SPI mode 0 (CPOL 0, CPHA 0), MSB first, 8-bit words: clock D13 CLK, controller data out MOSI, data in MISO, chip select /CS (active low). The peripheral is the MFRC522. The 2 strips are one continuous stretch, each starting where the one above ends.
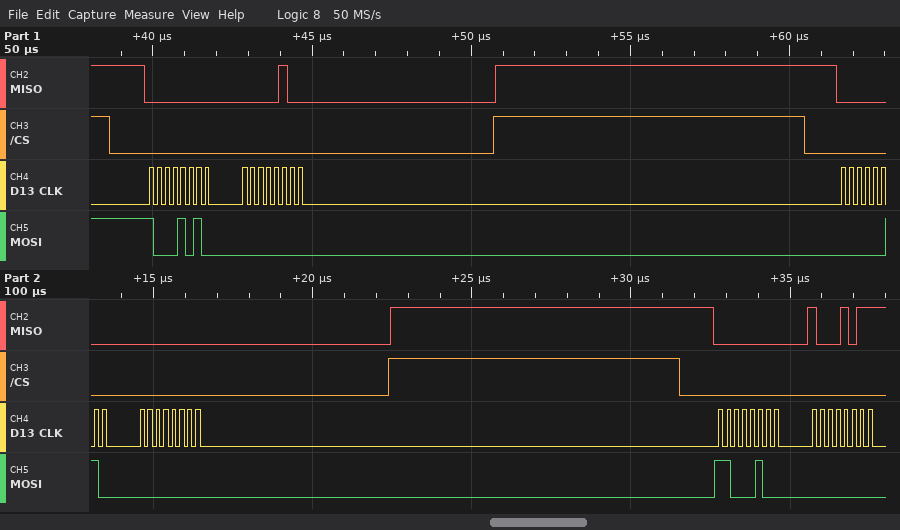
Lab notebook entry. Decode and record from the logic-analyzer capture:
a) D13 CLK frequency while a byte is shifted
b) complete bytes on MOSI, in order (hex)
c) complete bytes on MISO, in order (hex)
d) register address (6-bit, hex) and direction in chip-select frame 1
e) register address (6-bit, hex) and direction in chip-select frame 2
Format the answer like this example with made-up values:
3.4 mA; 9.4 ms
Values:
4 MHz; 8A 00 02 00 C4 00; 00 04 00 00 00 8B; 0x05 read; 0x01 write
